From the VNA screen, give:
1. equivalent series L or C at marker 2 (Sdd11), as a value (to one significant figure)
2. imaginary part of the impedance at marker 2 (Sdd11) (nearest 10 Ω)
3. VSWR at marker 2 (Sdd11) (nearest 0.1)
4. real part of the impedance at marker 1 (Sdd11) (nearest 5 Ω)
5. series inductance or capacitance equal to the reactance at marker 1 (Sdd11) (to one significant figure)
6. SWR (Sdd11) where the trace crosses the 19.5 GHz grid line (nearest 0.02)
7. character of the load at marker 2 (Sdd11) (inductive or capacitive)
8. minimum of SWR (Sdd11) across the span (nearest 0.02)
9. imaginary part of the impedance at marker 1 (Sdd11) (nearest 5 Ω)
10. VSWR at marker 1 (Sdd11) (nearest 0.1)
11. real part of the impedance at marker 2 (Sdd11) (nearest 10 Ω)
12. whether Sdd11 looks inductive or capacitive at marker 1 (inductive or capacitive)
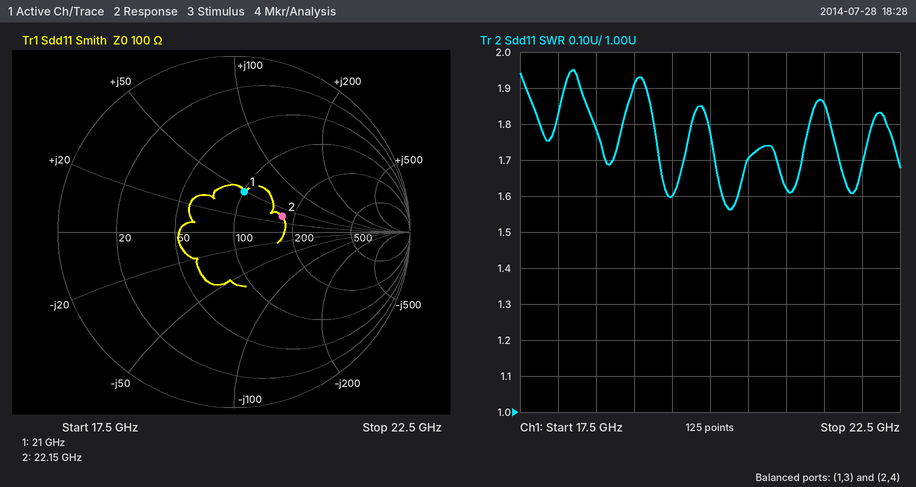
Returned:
200 pH
+30 Ω
1.8
100 Ω
400 pH
1.60
inductive
1.56
+50 Ω
1.6
170 Ω
inductive
